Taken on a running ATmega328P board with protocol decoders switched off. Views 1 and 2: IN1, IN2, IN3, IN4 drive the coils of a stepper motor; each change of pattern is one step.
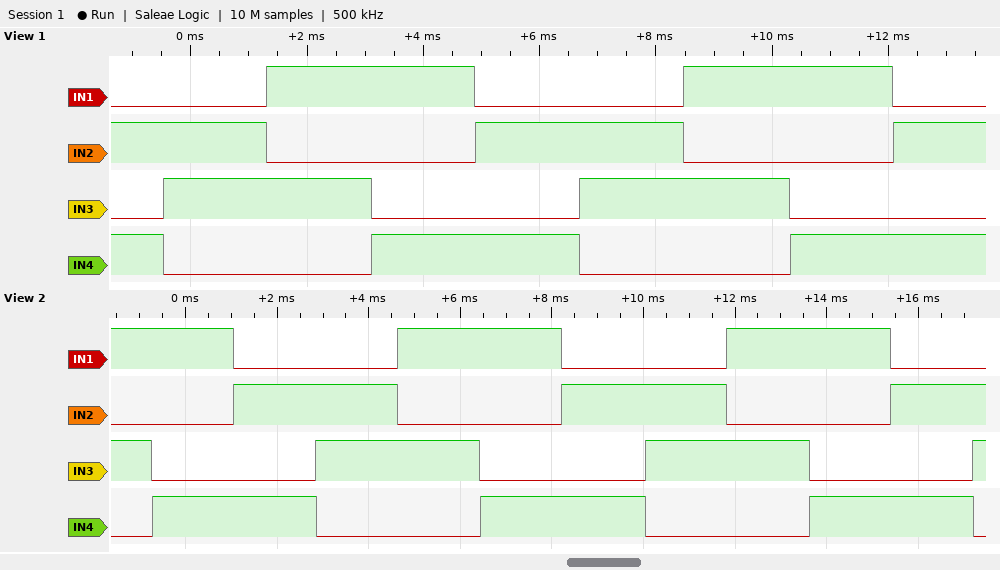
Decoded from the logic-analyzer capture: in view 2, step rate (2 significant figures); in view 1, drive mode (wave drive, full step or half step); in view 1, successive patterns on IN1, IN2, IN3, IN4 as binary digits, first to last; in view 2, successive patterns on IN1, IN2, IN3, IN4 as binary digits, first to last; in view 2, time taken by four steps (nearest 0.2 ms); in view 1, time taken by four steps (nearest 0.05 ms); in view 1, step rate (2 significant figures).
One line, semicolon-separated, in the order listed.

560 steps/s; full step; 0101 0110 1010 1001 0101 0110 1010 1001 0101; 1010 1001 0101 0110 1010 1001 0101 0110 1010 1001 0101 0110; 7.2 ms; 7.15 ms; 560 steps/s
